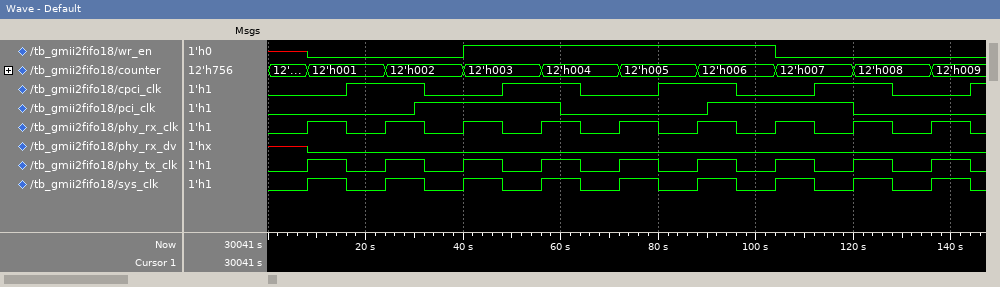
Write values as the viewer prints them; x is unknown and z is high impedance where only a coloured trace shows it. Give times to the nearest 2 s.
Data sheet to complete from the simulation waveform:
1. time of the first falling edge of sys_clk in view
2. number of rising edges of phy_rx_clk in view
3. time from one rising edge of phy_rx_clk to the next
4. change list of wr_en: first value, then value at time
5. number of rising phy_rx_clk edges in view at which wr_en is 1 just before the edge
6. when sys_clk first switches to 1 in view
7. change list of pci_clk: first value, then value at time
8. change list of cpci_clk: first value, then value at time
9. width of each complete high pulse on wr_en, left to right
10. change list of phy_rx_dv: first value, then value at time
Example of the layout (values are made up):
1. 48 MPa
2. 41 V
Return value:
1. 16 s
2. 9
3. 16 s
4. x, 0 at 8 s, 1 at 40 s, 0 at 104 s
5. 4
6. 8 s
7. 0, 1 at 30 s, 0 at 60 s, 1 at 90 s, 0 at 120 s
8. 0, 1 at 16 s, 0 at 32 s, 1 at 48 s, 0 at 64 s, 1 at 80 s, 0 at 96 s, 1 at 112 s, 0 at 128 s, 1 at 144 s
9. 64 s
10. x, 0 at 8 s
